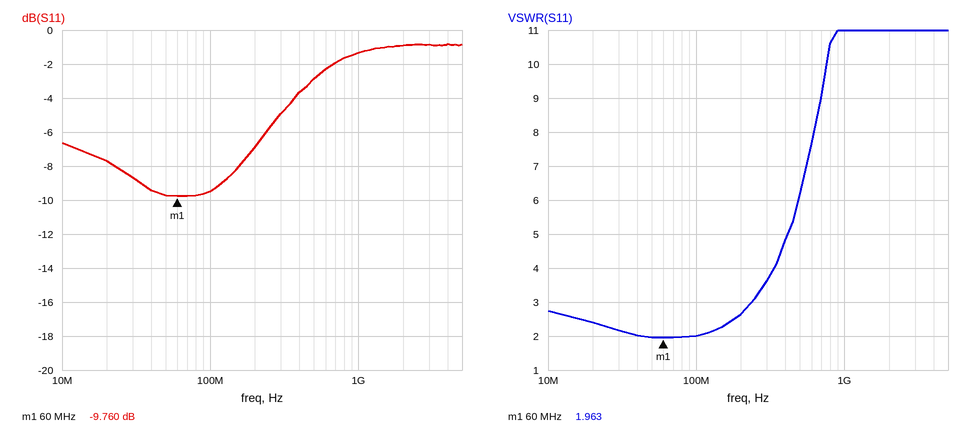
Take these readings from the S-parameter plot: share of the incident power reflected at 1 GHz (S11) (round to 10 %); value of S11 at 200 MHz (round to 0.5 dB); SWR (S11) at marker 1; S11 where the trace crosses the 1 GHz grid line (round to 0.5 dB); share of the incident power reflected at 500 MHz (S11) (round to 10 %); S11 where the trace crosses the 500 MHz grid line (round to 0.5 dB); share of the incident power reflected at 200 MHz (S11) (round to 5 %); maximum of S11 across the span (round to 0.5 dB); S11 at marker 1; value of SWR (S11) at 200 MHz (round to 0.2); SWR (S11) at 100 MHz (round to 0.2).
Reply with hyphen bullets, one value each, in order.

- 70 %
- -7.0 dB
- 1.963
- -1.5 dB
- 50 %
- -3.0 dB
- 20 %
- -1.0 dB
- -9.760 dB
- 2.6
- 2.0
